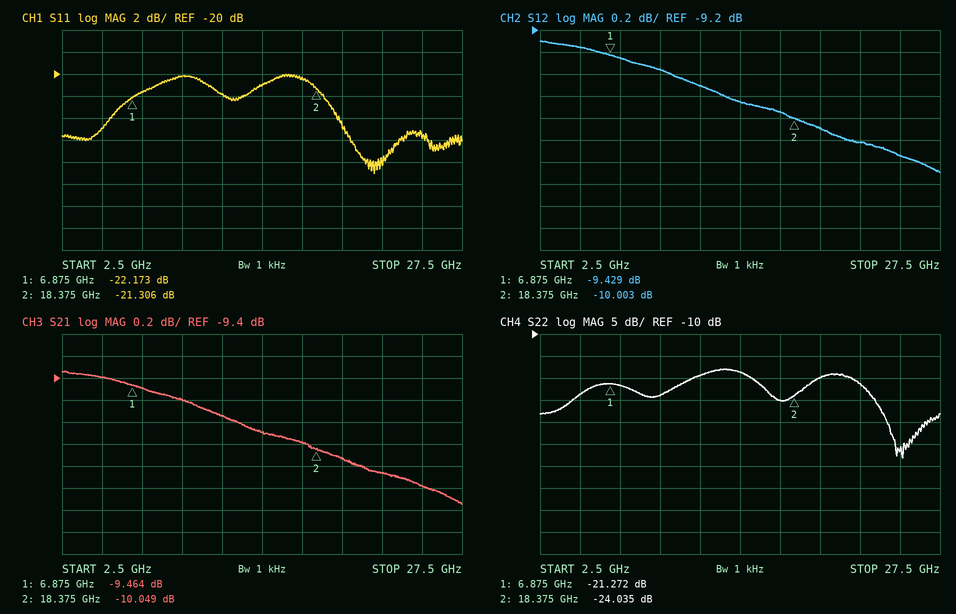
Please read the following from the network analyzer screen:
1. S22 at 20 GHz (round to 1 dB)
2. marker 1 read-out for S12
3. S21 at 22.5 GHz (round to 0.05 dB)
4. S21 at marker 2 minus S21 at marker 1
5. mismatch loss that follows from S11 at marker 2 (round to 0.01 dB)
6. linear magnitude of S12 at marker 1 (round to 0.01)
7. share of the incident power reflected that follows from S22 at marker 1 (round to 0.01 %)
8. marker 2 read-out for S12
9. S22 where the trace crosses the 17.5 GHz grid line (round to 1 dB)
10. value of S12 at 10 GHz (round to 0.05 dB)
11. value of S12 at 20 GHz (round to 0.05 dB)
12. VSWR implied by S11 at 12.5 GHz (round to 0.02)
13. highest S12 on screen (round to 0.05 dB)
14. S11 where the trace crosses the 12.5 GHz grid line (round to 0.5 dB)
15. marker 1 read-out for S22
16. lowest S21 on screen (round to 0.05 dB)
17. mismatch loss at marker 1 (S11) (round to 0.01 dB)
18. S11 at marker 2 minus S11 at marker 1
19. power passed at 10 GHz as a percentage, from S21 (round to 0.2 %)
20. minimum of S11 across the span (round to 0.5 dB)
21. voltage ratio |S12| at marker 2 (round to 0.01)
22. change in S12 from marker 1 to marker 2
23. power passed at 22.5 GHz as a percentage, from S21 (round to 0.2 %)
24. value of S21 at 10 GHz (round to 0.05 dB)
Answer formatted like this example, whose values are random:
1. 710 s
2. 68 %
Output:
1. -20 dB
2. -9.429 dB
3. -10.25 dB
4. -0.585 dB
5. 0.03 dB
6. 0.34
7. 0.75 %
8. -10.003 dB
9. -25 dB
10. -9.55 dB
11. -10.10 dB
12. 1.18
13. -9.30 dB
14. -22.0 dB
15. -21.272 dB
16. -10.55 dB
17. 0.03 dB
18. 0.867 dB
19. 11.0 %
20. -29.0 dB
21. 0.32
22. -0.574 dB
23. 9.4 %
24. -9.60 dB
